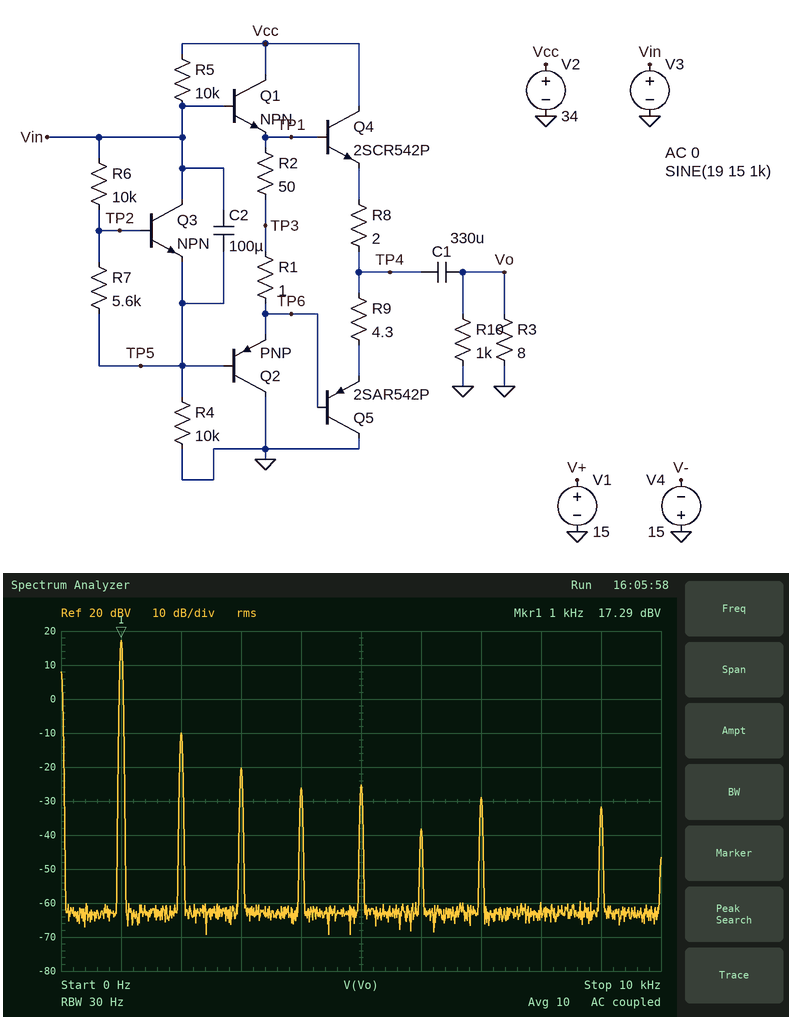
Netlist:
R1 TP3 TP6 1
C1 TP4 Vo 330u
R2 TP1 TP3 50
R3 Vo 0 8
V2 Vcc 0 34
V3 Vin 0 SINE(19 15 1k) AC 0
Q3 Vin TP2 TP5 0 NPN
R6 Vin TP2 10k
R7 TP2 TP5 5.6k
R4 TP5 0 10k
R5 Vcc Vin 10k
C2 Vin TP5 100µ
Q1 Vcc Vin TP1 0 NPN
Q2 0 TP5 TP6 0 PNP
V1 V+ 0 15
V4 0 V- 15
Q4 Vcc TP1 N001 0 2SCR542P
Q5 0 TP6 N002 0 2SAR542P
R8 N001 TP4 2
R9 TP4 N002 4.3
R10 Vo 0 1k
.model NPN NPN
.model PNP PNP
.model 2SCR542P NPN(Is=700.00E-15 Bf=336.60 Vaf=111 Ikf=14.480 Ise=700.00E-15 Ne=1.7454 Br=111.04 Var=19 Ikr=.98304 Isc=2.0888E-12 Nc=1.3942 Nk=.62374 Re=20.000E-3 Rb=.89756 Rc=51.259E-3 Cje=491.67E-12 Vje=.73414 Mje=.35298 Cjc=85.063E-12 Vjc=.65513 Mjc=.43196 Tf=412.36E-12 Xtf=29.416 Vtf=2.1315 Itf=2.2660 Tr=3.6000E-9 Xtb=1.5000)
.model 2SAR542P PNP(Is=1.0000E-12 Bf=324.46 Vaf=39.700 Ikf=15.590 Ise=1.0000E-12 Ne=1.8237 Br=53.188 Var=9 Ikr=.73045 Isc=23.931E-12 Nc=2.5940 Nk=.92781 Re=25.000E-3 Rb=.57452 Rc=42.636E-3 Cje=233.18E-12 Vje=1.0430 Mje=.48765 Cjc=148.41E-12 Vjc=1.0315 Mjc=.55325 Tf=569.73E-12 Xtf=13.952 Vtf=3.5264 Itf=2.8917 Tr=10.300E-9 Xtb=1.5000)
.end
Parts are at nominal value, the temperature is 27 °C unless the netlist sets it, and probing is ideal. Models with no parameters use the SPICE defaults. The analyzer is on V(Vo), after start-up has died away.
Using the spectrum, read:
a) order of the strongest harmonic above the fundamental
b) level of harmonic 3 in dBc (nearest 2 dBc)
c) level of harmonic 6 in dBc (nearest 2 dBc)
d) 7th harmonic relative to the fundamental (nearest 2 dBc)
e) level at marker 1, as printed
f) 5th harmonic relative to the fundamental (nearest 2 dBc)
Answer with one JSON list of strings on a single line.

["2", "-38 dBc", "-56 dBc", "-46 dBc", "17.29 dBV", "-42 dBc"]
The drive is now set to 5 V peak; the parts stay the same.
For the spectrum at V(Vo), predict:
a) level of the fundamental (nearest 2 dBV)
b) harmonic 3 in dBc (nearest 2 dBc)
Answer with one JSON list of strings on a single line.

["8 dBV", "-30 dBc"]
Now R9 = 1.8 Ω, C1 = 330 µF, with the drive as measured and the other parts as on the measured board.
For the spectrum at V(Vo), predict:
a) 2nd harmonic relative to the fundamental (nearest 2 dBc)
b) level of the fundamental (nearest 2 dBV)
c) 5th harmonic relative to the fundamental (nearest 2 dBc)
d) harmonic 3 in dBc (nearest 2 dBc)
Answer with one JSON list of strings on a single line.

["-48 dBc", "18 dBV", "-44 dBc", "-40 dBc"]
